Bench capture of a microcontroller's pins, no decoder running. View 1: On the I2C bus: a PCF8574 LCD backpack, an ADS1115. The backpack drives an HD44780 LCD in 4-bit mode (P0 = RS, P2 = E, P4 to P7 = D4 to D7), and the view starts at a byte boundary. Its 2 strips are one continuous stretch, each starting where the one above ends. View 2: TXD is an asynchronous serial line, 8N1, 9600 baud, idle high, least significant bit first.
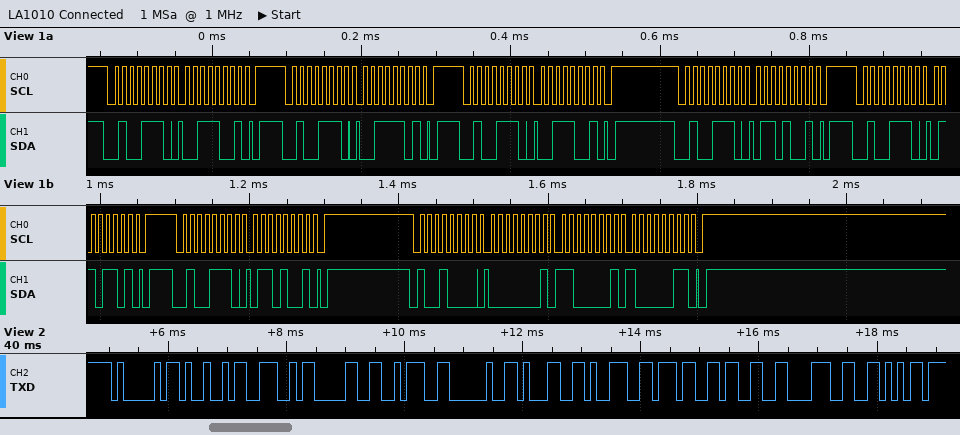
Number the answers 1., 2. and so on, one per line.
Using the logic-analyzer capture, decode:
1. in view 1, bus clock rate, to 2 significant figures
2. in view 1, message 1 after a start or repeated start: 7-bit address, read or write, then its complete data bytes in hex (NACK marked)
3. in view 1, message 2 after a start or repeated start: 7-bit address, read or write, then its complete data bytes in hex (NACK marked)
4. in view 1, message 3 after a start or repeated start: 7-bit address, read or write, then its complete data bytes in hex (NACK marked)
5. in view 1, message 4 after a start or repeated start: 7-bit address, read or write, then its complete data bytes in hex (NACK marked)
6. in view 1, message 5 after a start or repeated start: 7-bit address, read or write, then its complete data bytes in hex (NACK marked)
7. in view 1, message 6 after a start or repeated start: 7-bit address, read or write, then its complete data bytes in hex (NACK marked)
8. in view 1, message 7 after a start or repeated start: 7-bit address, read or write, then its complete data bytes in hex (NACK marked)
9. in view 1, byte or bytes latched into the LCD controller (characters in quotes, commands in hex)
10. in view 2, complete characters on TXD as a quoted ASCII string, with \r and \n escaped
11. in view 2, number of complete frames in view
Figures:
1. 100 kHz
2. 0x27 write: 39
3. 0x27 write: 3D
4. 0x27 write: 39
5. 0x27 write: 69
6. 0x27 write: 6D
7. 0x27 write: 69
8. 0x48 write: 01 C1 83
9. '6'
10. "AIN0: 19738V"
11. 12
